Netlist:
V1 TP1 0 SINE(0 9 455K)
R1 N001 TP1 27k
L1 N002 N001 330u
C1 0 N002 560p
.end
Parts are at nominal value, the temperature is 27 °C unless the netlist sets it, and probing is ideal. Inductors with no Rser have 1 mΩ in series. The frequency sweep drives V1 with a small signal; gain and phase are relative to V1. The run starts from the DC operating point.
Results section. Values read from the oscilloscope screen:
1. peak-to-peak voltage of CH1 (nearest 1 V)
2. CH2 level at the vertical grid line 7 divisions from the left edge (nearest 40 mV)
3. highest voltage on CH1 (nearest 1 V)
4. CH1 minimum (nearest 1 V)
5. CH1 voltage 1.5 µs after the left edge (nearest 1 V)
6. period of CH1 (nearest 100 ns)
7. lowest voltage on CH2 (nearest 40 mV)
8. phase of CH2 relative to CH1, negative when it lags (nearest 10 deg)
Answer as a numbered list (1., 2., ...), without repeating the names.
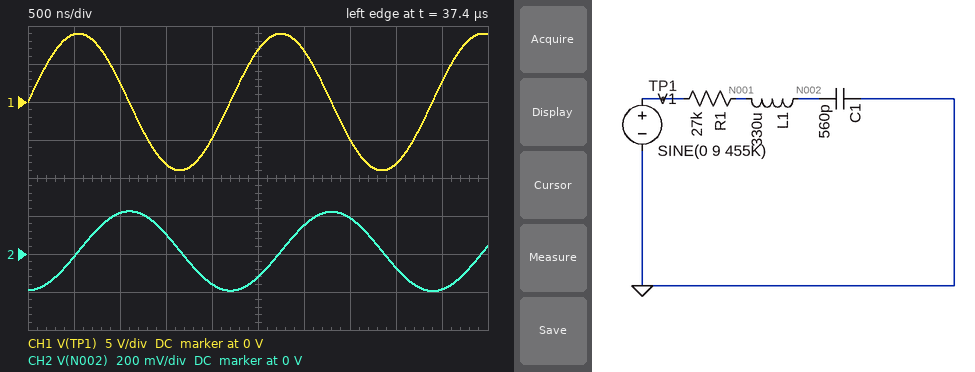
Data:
1. 18 V
2. 200 mV
3. 9 V
4. -9 V
5. -8 V
6. 2.2 µs
7. -200 mV
8. -90 deg
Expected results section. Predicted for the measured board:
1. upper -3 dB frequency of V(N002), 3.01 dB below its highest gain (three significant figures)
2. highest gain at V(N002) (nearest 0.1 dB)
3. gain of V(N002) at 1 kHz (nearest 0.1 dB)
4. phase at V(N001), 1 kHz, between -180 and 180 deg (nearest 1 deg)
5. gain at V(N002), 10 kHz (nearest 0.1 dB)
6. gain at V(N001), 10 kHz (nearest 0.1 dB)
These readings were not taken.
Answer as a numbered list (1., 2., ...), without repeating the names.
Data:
1. 10.5 kHz
2. 0 dB
3. 0 dB
4. -5 deg
5. -2.8 dB
6. -2.8 dB
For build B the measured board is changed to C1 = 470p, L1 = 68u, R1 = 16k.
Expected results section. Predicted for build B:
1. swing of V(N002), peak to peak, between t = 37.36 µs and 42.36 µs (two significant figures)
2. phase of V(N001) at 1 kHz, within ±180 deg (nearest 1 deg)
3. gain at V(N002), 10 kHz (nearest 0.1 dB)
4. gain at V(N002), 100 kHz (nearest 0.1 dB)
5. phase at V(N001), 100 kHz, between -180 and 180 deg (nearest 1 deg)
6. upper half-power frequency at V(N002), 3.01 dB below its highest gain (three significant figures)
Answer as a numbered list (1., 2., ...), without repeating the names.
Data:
1. 840 mV
2. -3 deg
3. -0.9 dB
4. -13.7 dB
5. -78 deg
6. 21.2 kHz
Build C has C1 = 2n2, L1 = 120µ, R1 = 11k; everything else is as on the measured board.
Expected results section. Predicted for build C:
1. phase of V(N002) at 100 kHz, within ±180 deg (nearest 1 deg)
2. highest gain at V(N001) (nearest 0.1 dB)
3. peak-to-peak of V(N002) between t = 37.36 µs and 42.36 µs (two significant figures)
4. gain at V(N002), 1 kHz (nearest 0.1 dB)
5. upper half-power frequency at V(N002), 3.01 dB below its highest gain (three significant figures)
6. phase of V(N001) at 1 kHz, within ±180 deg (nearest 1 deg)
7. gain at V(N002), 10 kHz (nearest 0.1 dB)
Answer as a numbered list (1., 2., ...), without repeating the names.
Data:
1. -87 deg
2. 0 dB
3. 260 mV
4. -0.1 dB
5. 6.58 kHz
6. -9 deg
7. -5.2 dB
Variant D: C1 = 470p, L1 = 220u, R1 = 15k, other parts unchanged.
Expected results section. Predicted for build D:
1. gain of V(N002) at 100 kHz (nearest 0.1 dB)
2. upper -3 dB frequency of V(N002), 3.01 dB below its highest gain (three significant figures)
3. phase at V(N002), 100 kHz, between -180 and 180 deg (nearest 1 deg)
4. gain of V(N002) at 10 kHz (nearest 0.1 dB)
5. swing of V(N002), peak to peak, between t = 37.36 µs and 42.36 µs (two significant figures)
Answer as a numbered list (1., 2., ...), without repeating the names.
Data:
1. -13.1 dB
2. 22.6 kHz
3. -78 deg
4. -0.8 dB
5. 890 mV
